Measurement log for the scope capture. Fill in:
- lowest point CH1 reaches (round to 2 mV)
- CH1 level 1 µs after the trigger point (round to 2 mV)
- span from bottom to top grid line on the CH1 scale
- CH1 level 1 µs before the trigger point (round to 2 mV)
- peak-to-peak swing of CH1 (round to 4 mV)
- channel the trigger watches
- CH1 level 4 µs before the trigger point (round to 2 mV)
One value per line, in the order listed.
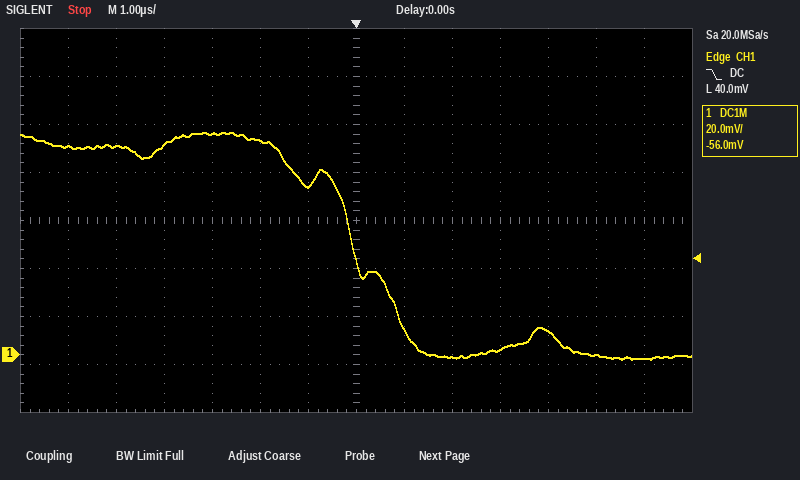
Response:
-2 mV
10 mV
160 mV
70 mV
96 mV
CH1
88 mV
